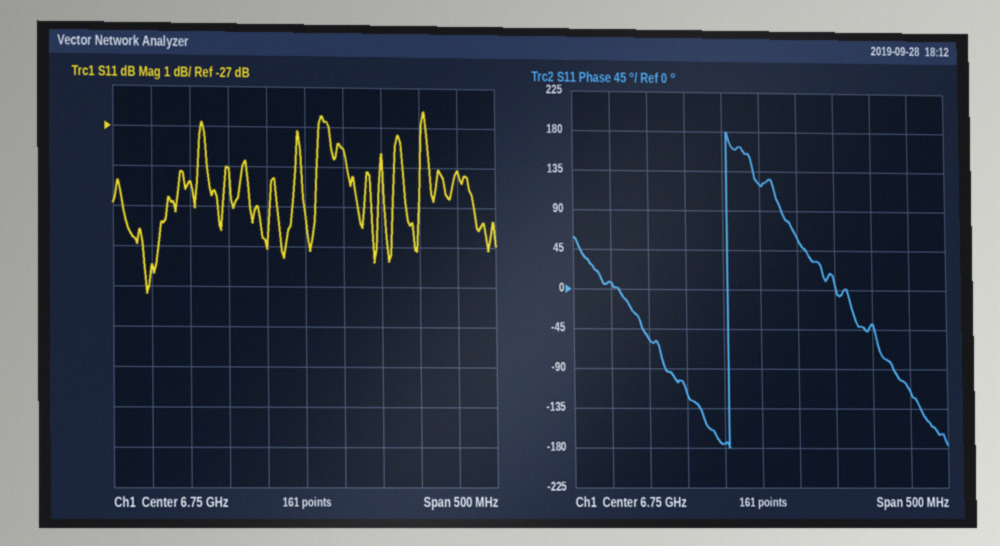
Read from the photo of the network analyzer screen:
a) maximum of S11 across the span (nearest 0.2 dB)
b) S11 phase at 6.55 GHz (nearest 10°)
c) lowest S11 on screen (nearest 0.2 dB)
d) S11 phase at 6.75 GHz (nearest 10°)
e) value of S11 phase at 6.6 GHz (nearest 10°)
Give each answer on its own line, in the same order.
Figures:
-26.6 dB
10°
-31.2 dB
120°
-60°
